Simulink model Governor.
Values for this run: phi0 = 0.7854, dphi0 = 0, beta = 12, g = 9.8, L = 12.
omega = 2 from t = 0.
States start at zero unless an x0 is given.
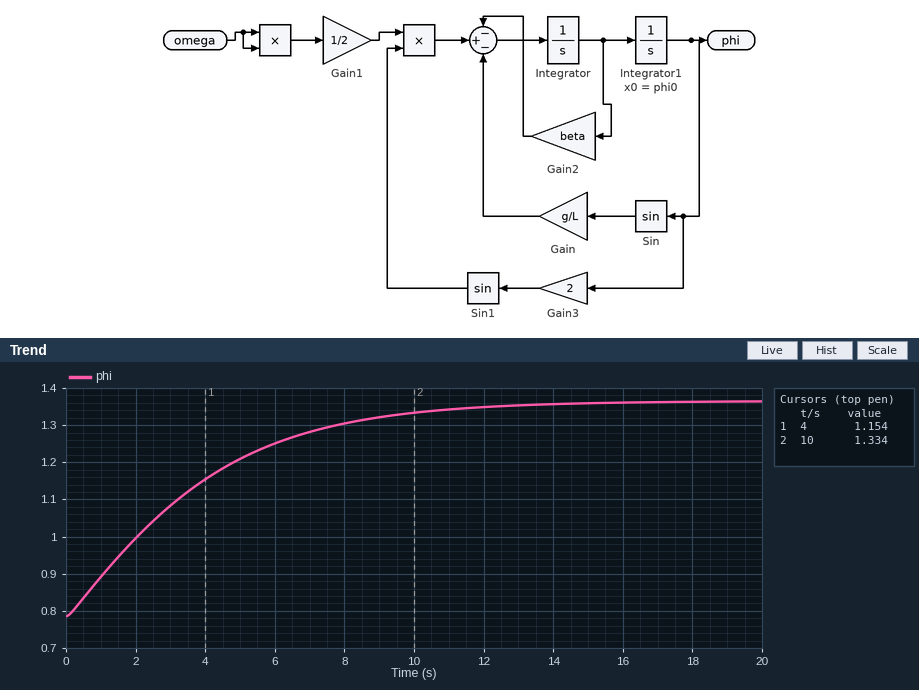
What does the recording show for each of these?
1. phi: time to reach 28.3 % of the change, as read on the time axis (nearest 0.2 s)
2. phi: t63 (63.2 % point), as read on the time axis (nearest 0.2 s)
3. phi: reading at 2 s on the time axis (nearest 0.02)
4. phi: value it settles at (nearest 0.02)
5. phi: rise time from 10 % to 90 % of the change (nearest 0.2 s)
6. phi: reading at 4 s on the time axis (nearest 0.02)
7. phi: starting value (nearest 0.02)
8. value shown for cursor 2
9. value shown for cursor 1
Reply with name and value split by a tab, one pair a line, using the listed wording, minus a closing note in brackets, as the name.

phi: time to reach 28.3 % of the change, as read on the time axis	1.6 s
phi: t63 (63.2 % point), as read on the time axis	4.0 s
phi: reading at 2 s on the time axis	1.00
phi: value it settles at	1.36
phi: rise time from 10 % to 90 % of the change	7.6 s
phi: reading at 4 s on the time axis	1.16
phi: starting value	0.78
value shown for cursor 2	1.334
value shown for cursor 1	1.154
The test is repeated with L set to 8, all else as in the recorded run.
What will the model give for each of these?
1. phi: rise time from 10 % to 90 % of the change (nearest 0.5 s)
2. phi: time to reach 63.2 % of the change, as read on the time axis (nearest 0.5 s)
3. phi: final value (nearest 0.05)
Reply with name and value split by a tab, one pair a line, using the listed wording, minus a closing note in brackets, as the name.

phi: rise time from 10 % to 90 % of the change	8.0 s
phi: time to reach 63.2 % of the change, as read on the time axis	4.0 s
phi: final value	1.25
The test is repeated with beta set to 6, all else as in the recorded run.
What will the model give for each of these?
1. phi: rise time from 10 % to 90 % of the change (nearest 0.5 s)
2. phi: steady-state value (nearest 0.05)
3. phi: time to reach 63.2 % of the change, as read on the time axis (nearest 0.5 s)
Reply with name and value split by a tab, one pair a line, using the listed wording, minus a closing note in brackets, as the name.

phi: rise time from 10 % to 90 % of the change	3.5 s
phi: steady-state value	1.35
phi: time to reach 63.2 % of the change, as read on the time axis	2.0 s
